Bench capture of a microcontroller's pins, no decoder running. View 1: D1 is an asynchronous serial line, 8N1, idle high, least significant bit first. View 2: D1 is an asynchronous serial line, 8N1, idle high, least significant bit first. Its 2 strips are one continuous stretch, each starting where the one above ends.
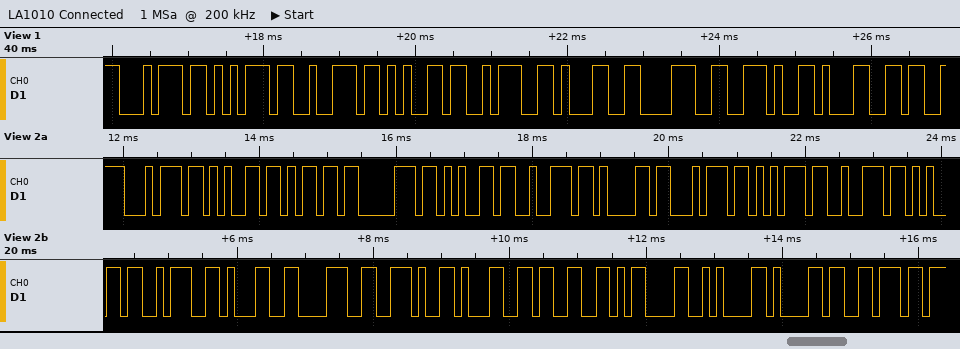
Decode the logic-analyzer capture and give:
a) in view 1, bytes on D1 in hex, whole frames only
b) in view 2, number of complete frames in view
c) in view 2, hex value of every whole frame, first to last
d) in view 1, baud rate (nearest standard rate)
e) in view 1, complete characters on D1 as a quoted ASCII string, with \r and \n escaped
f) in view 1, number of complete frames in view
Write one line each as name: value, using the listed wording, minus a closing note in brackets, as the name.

in view 1, bytes on D1 in hex, whole frames only: 74 75 72 65 3A 31 38 2E 31
in view 2, number of complete frames in view: 21
in view 2, hex value of every whole frame, first to last: 74 65 6D 70 65 72 61 74 75 72 65 3A 31 38 2E 31 33 0D 0A 61 76
in view 1, baud rate: 9600 baud
in view 1, complete characters on D1 as a quoted ASCII string, with \r and \n escaped: "ture:18.1"
in view 1, number of complete frames in view: 9
